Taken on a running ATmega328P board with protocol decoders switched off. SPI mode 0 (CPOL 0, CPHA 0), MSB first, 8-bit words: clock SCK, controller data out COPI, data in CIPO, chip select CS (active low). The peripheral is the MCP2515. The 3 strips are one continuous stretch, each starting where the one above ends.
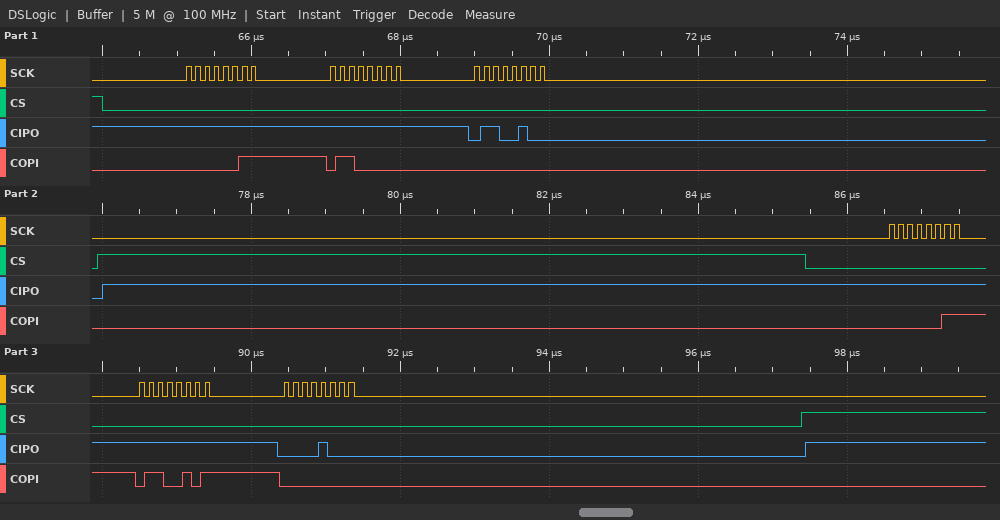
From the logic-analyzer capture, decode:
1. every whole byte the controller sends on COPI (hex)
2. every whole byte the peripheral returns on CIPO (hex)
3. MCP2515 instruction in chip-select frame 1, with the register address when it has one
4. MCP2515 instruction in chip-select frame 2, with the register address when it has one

03 60 00 03 65 00
FF FF 64 FF FF 08
READ 0x60
READ 0x65
